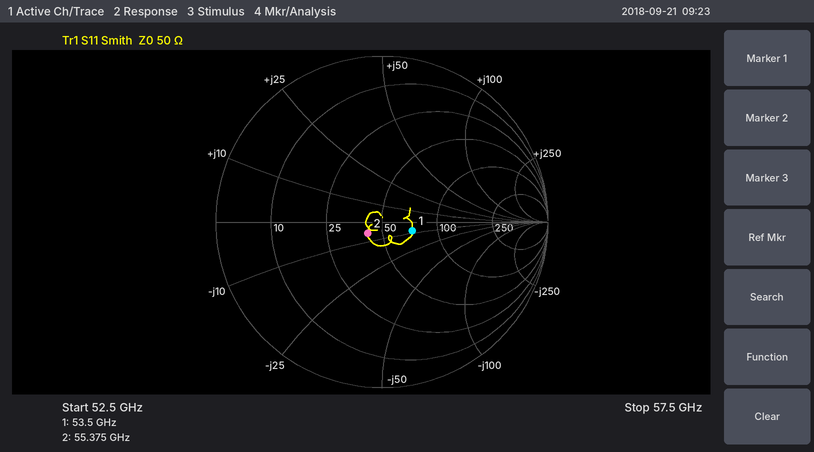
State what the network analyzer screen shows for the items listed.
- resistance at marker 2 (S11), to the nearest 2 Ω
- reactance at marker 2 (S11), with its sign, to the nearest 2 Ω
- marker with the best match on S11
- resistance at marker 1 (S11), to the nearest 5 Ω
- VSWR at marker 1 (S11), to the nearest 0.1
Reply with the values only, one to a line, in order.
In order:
42 Ω
-6 Ω
marker 2
70 Ω
1.5
